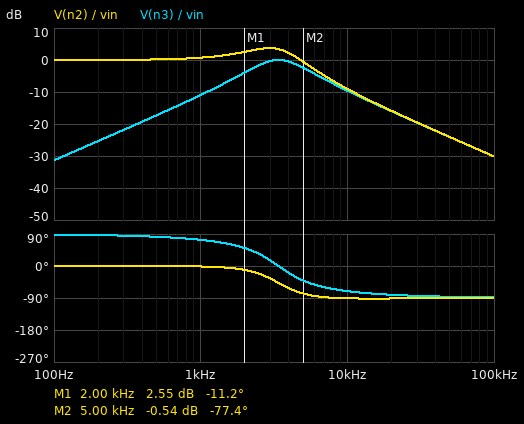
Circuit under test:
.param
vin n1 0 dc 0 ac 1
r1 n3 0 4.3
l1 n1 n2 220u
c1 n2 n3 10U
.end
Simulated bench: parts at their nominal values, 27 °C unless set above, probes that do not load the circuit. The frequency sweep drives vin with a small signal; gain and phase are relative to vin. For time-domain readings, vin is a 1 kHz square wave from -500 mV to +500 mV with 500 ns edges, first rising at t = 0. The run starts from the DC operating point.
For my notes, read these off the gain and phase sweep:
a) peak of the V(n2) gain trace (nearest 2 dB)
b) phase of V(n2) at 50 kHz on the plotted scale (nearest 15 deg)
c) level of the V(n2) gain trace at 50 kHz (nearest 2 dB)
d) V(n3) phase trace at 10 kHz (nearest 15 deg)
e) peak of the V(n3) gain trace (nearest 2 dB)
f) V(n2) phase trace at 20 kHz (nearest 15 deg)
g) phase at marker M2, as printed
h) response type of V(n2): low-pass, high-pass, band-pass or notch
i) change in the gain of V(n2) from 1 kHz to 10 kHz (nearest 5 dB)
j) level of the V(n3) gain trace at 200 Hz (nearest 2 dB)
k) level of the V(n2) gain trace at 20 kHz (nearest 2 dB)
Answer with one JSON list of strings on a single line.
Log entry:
["4 dB", "-90 deg", "-24 dB", "-75 deg", "0 dB", "-90 deg", "-77.4 deg", "low-pass", "-10 dB", "-26 dB", "-16 dB"]
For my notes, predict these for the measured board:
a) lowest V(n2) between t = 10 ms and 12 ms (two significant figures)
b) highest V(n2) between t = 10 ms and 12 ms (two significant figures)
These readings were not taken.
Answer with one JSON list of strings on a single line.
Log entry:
["-830 mV", "830 mV"]
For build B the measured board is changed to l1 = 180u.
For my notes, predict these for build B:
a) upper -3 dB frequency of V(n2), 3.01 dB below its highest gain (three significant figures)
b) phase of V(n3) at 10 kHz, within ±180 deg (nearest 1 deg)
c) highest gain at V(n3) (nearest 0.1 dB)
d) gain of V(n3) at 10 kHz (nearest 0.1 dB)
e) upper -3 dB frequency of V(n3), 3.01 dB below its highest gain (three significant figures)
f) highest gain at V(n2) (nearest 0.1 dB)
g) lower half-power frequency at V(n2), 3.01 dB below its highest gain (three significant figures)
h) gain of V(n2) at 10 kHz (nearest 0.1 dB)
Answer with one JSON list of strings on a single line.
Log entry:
["5.18 kHz", "-66 deg", "0 dB", "-7.9 dB", "6.11 kHz", "3.3 dB", "663 Hz", "-7.3 dB"]
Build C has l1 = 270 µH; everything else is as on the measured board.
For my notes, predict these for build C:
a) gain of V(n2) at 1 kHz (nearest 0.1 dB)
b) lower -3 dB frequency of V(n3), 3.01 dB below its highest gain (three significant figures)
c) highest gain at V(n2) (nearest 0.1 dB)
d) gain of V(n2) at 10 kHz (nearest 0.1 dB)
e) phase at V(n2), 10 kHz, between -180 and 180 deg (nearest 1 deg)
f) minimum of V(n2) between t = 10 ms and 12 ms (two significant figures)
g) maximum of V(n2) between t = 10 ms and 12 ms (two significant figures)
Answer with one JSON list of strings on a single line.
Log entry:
["0.9 dB", "2.05 kHz", "4.2 dB", "-10.8 dB", "-95 deg", "-860 mV", "860 mV"]
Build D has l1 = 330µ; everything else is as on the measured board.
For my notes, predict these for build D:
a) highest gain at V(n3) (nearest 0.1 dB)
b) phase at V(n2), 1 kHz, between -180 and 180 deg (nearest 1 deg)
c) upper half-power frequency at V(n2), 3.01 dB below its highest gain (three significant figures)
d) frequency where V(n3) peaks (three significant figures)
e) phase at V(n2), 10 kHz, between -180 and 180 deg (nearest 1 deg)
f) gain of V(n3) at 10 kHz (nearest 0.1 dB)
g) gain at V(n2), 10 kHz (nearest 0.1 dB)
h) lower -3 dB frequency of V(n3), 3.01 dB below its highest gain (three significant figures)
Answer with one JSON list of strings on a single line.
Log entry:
["0 dB", "-2 deg", "3.52 kHz", "2.77 kHz", "-98 deg", "-13.2 dB", "-12.6 dB", "1.92 kHz"]
